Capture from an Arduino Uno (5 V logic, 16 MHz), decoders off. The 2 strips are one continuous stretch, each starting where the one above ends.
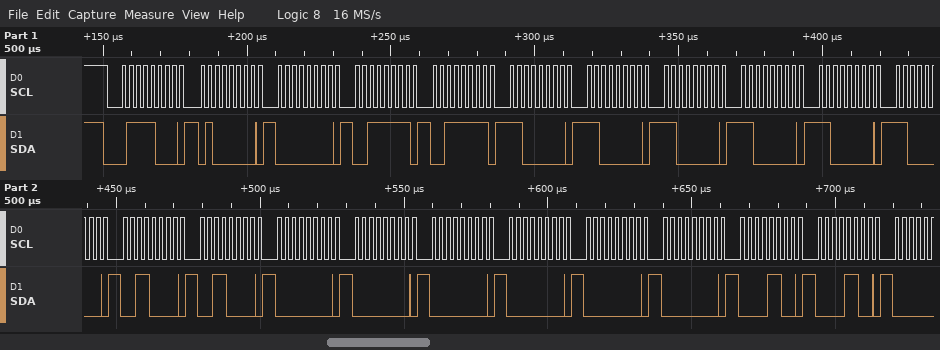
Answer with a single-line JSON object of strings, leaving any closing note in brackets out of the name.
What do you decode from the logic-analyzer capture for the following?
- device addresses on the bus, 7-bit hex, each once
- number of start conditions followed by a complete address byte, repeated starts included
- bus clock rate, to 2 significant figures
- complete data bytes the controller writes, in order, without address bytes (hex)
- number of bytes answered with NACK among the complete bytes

{"device addresses on the bus, 7-bit hex, each once": "0x3C", "number of start conditions followed by a complete address byte, repeated starts included": "1", "bus clock rate, to 2 significant figures": "400 kHz", "complete data bytes the controller writes, in order, without address bytes": "40 00 3F 3F C0 C0 C0 C0 C0 C0 30 30 00 00 00 00 00 00 0C 0C", "number of bytes answered with NACK among the complete bytes": "0"}
